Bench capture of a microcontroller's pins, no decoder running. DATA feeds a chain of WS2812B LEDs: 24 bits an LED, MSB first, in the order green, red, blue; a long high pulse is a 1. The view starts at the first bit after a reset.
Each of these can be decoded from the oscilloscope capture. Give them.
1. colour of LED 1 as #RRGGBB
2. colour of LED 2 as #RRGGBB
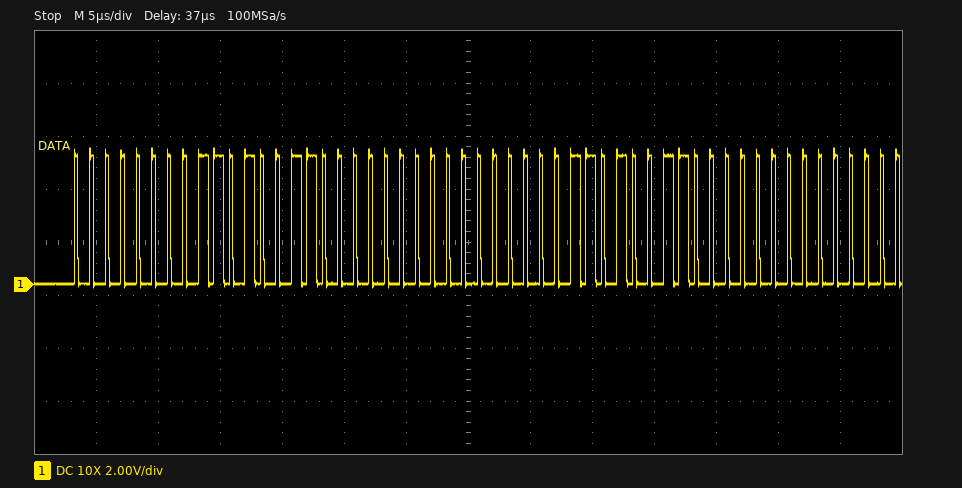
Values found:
#D30000
#D30000
